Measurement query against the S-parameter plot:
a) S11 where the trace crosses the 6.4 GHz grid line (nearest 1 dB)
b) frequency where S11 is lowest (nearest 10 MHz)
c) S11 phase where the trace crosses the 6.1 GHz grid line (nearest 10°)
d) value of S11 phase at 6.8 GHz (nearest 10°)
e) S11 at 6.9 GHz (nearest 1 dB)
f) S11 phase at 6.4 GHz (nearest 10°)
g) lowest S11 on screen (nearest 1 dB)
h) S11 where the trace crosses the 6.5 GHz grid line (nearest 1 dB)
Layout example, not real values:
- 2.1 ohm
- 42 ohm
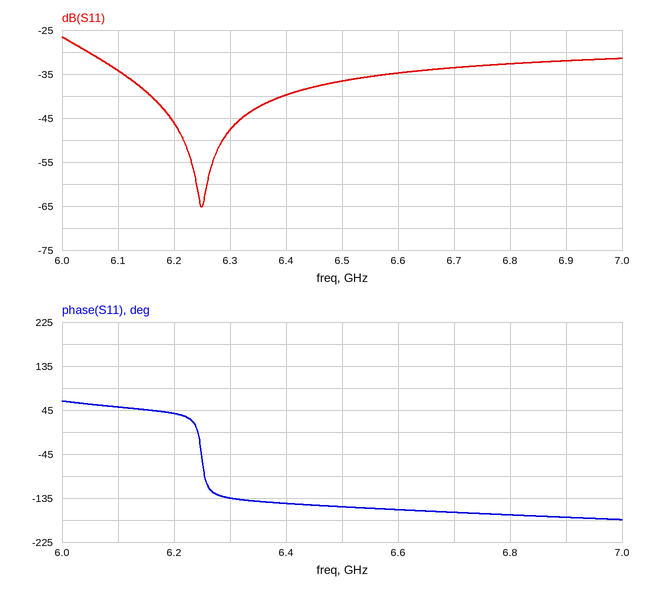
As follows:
- -40 dB
- 6.25 GHz
- 50°
- -170°
- -32 dB
- -150°
- -65 dB
- -37 dB
